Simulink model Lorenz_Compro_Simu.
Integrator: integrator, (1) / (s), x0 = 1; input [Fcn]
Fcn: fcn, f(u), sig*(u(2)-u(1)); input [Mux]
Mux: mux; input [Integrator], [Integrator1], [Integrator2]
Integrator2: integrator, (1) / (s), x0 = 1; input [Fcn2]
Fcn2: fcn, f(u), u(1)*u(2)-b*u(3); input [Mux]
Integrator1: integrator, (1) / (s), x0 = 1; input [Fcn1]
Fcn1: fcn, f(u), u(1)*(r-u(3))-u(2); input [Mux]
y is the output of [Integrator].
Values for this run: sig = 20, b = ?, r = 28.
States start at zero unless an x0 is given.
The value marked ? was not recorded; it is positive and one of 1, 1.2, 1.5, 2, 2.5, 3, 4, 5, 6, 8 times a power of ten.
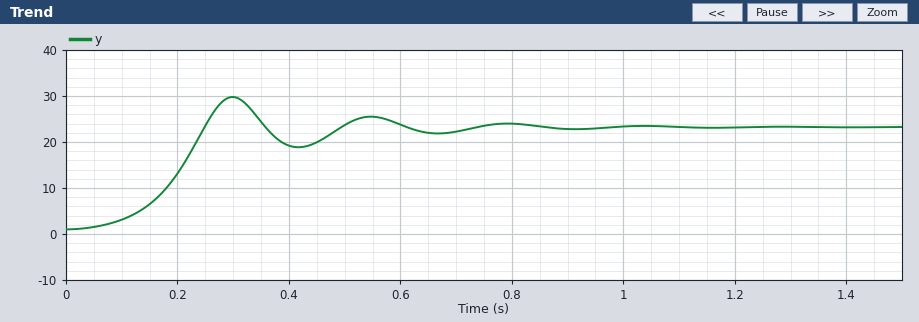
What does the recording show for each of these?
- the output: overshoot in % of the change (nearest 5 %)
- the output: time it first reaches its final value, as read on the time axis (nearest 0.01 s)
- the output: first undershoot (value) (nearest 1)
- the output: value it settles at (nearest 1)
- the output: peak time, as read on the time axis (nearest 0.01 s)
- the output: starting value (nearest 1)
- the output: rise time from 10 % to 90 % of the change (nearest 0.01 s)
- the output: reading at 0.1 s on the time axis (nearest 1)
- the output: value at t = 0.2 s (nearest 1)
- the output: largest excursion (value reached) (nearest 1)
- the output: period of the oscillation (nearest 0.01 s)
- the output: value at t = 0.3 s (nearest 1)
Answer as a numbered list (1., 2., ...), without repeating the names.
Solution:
1. 30 %
2. 0.25 s
3. 19
4. 23
5. 0.30 s
6. 1
7. 0.14 s
8. 3
9. 13
10. 30
11. 0.25 s
12. 30
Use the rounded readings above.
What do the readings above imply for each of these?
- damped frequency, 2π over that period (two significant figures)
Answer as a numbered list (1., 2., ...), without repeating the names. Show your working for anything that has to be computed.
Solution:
1. 2π / 0.25 = 25 rad/s
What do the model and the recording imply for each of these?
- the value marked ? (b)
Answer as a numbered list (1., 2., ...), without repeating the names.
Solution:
1. 20
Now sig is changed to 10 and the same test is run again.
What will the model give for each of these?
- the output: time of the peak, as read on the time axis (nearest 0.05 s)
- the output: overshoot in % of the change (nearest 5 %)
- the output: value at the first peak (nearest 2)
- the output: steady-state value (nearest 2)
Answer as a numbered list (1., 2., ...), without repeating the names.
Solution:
1. 0.40 s
2. 20 %
3. 28
4. 24
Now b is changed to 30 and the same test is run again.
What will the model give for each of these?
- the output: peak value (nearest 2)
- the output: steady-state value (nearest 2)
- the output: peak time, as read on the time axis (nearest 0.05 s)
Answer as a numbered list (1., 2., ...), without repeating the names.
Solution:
1. 34
2. 28
3. 0.30 s
